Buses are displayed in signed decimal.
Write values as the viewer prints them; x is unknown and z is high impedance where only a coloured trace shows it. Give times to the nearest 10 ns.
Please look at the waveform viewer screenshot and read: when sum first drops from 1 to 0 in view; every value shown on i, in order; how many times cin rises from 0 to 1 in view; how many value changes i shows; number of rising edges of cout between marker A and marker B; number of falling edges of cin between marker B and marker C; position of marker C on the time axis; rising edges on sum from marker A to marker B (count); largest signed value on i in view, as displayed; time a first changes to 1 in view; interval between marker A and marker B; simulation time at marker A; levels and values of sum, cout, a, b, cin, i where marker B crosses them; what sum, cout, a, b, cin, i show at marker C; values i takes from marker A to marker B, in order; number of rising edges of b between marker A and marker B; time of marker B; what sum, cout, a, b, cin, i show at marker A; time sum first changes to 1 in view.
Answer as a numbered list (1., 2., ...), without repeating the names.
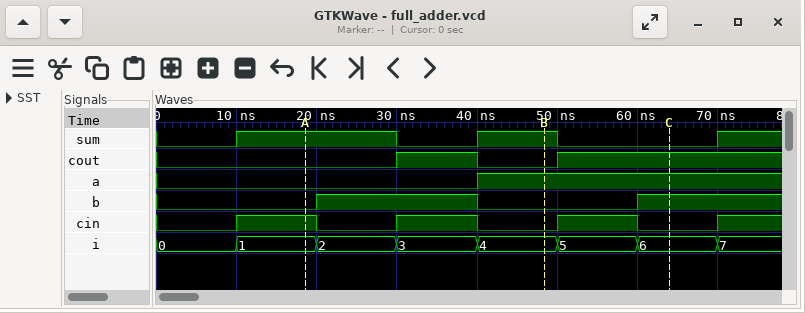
1. 30 ns
2. 0, 1, 2, 3, 4, 5, 6, 7
3. 4
4. 7
5. 1
6. 1
7. 60 ns
8. 1
9. 7
10. 40 ns
11. 30 ns
12. 20 ns
13. sum=1, cout=0, a=1, b=0, cin=0, i=4
14. sum=0, cout=1, a=1, b=1, cin=0, i=6
15. 1, 2, 3, 4
16. 1
17. 50 ns
18. sum=1, cout=0, a=0, b=0, cin=1, i=1
19. 10 ns
